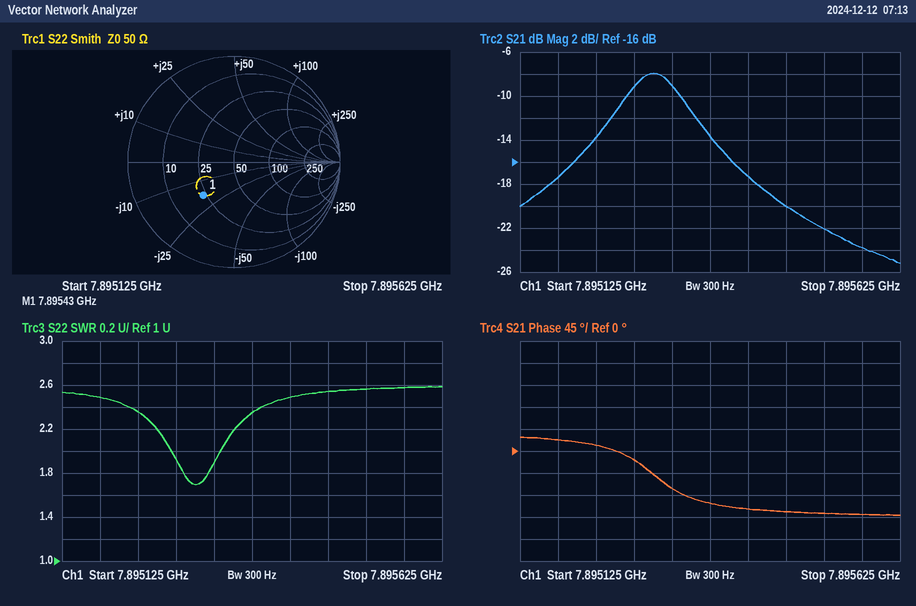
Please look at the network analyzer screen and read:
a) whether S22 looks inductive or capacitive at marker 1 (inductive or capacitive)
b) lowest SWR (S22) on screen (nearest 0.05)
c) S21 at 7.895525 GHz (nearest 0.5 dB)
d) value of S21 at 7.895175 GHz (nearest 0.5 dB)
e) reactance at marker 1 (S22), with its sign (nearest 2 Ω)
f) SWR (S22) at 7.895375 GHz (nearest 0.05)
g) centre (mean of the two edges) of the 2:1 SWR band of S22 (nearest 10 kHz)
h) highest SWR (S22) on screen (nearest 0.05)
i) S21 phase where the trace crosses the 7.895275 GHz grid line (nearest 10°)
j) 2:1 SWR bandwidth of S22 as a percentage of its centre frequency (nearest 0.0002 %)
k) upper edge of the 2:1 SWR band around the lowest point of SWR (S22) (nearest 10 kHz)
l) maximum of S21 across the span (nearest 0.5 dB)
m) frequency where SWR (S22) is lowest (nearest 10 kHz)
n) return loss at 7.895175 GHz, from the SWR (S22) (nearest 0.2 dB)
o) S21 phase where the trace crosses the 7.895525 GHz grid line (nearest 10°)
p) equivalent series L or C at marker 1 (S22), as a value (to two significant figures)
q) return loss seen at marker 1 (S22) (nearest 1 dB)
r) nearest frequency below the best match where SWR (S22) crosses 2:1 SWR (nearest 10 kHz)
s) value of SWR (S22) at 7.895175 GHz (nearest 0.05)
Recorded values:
capacitive
1.70
-22.0 dB
-17.5 dB
-18 Ω
2.35
7.89530 GHz
2.60
-20°
0.0008 %
7.89533 GHz
-8.0 dB
7.89530 GHz
7.4 dB
-130°
1.1 pF
7 dB
7.89527 GHz
2.50
